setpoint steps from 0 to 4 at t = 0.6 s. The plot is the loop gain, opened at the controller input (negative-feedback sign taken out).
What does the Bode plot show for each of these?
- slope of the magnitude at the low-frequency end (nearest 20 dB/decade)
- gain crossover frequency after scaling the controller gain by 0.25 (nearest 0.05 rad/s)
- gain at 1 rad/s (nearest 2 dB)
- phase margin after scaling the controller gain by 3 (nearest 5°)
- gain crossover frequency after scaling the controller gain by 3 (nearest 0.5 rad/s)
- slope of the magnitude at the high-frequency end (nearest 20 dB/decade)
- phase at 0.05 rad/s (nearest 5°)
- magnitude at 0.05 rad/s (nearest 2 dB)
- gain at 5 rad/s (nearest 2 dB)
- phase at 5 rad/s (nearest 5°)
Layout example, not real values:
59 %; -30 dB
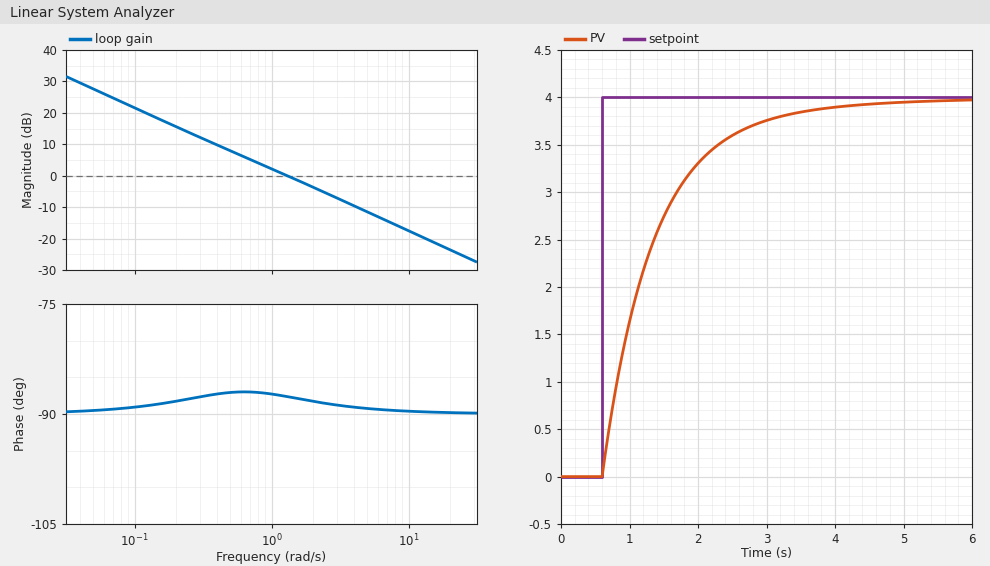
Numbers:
-20 dB/decade; 0.30 rad/s; 2 dB; 90°; 4.0 rad/s; -20 dB/decade; -90°; 28 dB; -12 dB; -90°
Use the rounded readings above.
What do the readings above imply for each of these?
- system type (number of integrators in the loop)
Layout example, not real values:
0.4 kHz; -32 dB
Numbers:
1
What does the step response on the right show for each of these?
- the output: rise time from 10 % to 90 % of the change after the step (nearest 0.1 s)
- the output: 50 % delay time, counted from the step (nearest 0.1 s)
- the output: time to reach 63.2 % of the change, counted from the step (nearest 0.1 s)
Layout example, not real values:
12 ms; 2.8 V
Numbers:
1.8 s; 0.5 s; 0.8 s
